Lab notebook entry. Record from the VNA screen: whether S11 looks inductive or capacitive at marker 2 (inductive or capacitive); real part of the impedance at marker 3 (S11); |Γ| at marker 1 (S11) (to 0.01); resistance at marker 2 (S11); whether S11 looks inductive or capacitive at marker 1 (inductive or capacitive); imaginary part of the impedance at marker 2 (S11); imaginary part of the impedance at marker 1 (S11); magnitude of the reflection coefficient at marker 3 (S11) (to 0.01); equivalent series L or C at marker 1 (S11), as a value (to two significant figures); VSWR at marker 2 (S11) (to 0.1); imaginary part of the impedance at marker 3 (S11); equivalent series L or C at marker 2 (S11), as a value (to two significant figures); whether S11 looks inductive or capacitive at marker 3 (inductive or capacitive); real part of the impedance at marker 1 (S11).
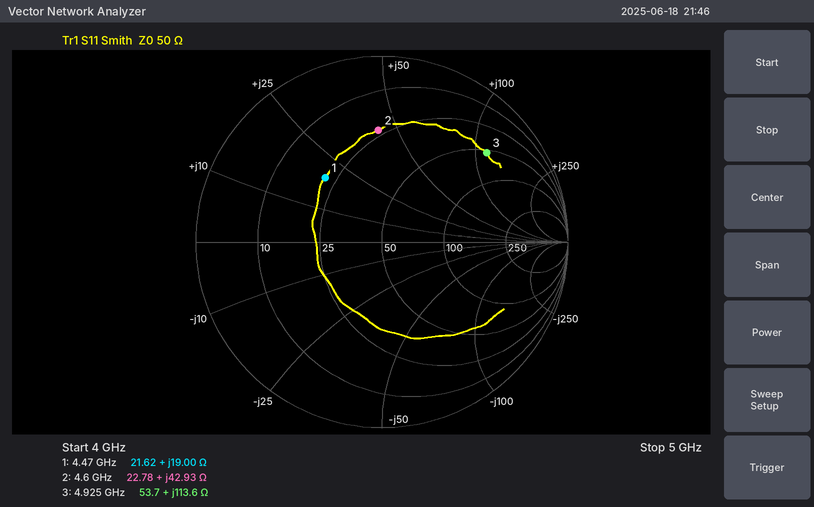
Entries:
inductive
53.7 Ω
0.46
22.78 Ω
inductive
+42.93 Ω
+19.00 Ω
0.74
680 pH
4.0
+113.6 Ω
1.5 nH
inductive
21.62 Ω
